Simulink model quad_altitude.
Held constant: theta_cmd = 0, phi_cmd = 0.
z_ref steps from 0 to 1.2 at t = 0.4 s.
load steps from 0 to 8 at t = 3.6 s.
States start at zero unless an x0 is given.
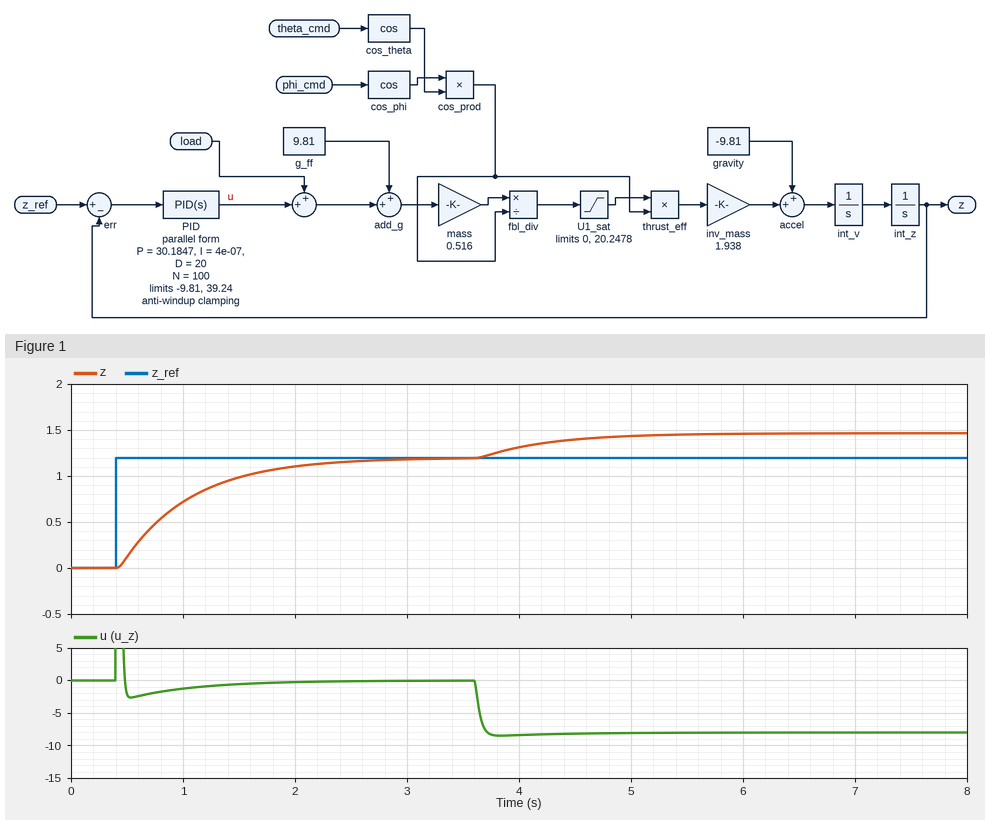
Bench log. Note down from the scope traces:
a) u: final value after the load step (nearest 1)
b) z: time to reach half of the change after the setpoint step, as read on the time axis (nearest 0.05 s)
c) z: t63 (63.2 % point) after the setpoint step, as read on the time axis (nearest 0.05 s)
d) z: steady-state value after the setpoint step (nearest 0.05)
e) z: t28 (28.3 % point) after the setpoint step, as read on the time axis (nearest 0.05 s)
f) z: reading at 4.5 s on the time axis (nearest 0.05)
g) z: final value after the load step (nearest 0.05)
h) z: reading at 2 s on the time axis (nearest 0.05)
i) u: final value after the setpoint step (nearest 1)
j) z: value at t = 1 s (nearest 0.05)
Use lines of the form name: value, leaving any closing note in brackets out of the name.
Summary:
u: final value after the load step: -8
z: time to reach half of the change after the setpoint step, as read on the time axis: 0.85 s
z: t63 (63.2 % point) after the setpoint step, as read on the time axis: 1.05 s
z: steady-state value after the setpoint step: 1.20
z: t28 (28.3 % point) after the setpoint step, as read on the time axis: 0.65 s
z: reading at 4.5 s on the time axis: 1.40
z: final value after the load step: 1.45
z: reading at 2 s on the time axis: 1.10
u: final value after the setpoint step: 0
z: value at t = 1 s: 0.70
